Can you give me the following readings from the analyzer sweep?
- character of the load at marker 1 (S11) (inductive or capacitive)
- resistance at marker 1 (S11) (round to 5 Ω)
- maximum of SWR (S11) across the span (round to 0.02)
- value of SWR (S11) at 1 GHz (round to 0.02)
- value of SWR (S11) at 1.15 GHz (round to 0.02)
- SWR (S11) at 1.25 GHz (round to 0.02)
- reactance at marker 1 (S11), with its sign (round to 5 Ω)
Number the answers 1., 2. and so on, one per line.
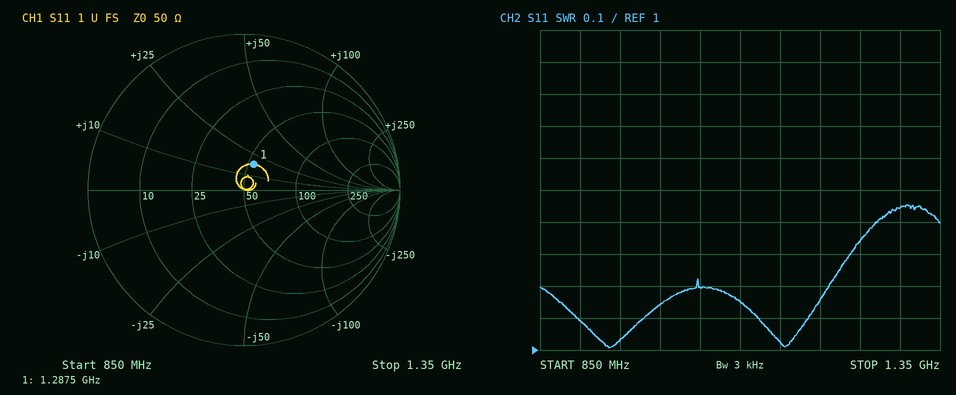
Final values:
1. inductive
2. 55 Ω
3. 1.46
4. 1.14
5. 1.02
6. 1.34
7. +20 Ω
